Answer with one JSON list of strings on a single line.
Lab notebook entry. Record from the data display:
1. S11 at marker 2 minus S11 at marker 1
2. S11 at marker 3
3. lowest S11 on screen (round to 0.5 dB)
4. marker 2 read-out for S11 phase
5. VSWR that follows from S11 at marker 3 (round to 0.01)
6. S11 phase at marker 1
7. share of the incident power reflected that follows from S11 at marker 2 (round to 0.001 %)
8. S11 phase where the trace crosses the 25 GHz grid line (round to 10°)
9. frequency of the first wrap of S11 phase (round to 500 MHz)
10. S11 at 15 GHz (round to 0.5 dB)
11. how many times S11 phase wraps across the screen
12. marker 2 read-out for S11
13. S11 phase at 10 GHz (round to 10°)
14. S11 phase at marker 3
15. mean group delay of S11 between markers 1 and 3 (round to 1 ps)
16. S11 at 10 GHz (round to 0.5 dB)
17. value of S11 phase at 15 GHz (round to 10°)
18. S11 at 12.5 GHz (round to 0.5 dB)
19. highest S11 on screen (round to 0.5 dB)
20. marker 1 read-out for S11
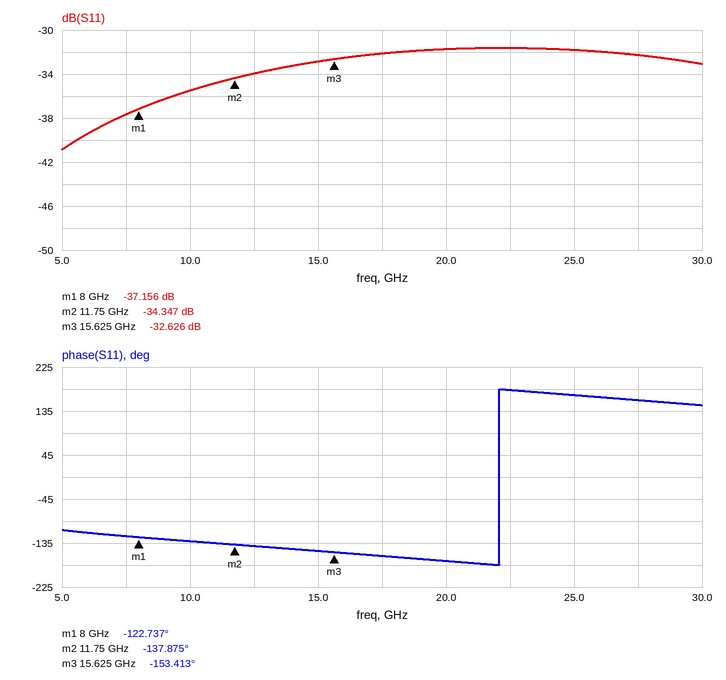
["2.809 dB", "-32.626 dB", "-41.0 dB", "-137.875°", "1.05", "-122.737°", "0.037 %", "170°", "22.0 GHz", "-33.0 dB", "1", "-34.347 dB", "-130°", "-153.413°", "11 ps", "-35.5 dB", "-150°", "-34.0 dB", "-31.5 dB", "-37.156 dB"]
